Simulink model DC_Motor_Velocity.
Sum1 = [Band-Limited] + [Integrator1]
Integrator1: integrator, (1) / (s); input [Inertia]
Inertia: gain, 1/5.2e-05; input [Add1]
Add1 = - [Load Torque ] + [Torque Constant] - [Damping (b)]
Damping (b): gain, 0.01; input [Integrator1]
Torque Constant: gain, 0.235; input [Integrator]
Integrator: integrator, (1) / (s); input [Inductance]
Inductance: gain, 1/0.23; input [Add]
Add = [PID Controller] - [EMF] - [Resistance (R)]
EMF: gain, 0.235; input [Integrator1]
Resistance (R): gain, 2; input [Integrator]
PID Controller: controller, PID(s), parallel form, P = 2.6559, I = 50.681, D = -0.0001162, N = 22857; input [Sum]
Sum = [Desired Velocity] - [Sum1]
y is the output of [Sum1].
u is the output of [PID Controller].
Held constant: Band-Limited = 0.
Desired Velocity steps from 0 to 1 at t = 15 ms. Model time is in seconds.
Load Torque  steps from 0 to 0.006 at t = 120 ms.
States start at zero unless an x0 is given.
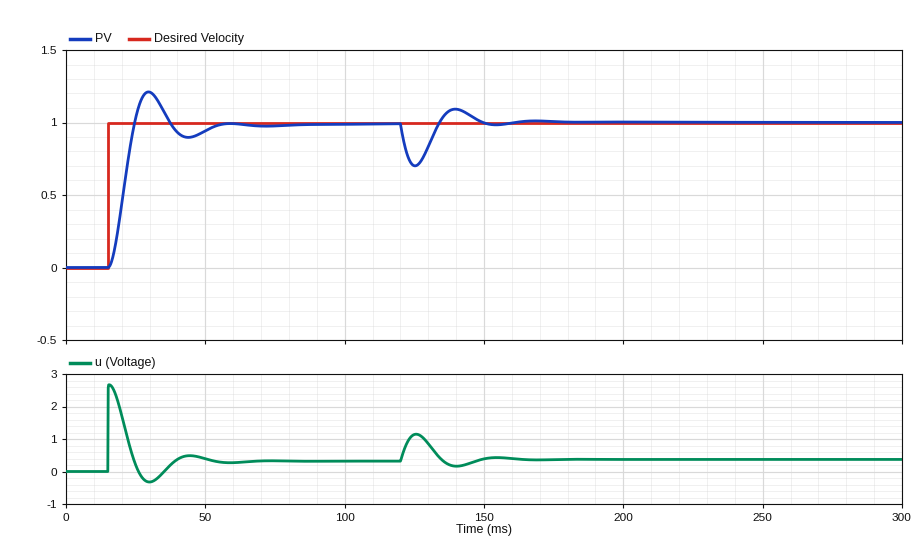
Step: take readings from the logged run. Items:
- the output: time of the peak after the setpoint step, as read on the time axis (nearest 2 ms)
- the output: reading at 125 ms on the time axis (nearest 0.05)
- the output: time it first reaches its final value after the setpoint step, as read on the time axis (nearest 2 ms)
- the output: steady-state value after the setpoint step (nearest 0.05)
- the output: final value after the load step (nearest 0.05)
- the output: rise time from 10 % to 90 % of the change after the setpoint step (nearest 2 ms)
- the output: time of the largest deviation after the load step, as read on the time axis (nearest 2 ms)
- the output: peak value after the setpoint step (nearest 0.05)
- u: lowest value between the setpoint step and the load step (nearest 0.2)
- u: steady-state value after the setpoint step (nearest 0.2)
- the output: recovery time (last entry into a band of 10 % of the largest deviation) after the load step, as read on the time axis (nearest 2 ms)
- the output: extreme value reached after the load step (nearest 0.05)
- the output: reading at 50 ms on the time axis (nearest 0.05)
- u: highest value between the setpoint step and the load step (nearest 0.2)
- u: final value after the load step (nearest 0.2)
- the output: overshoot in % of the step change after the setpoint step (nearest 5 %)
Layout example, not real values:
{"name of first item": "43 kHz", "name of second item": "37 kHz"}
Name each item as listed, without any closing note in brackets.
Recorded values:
{"the output: time of the peak after the setpoint step, as read on the time axis": "30 ms", "the output: reading at 125 ms on the time axis": "0.70", "the output: time it first reaches its final value after the setpoint step, as read on the time axis": "24 ms", "the output: steady-state value after the setpoint step": "1.00", "the output: final value after the load step": "1.00", "the output: rise time from 10 % to 90 % of the change after the setpoint step": "6 ms", "the output: time of the largest deviation after the load step, as read on the time axis": "126 ms", "the output: peak value after the setpoint step": "1.20", "u: lowest value between the setpoint step and the load step": "-0.4", "u: steady-state value after the setpoint step": "0.4", "the output: recovery time (last entry into a band of 10 % of the largest deviation) after the load step, as read on the time axis": "146 ms", "the output: extreme value reached after the load step": "0.70", "the output: reading at 50 ms on the time axis": "0.95", "u: highest value between the setpoint step and the load step": "2.6", "u: final value after the load step": "0.4", "the output: overshoot in % of the step change after the setpoint step": "20 %"}
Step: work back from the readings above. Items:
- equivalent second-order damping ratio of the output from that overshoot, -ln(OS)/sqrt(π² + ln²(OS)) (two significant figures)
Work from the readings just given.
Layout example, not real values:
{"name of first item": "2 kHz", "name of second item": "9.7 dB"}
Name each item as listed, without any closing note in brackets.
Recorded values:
{"equivalent second-order damping ratio of the output from that overshoot, -ln(OS)/sqrt(π² + ln²(OS))": "0.46"}
